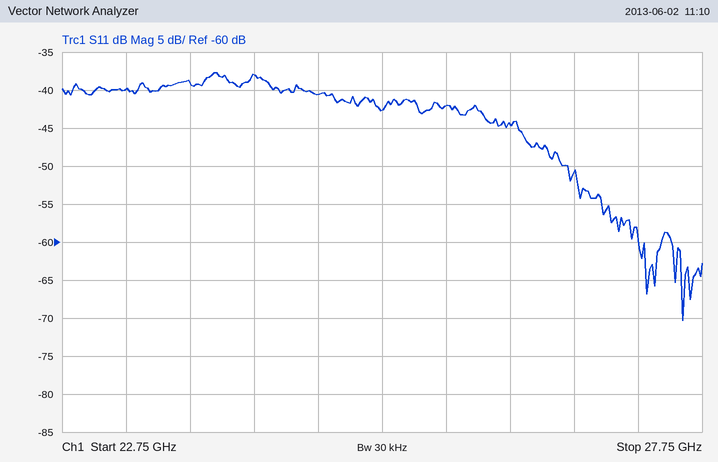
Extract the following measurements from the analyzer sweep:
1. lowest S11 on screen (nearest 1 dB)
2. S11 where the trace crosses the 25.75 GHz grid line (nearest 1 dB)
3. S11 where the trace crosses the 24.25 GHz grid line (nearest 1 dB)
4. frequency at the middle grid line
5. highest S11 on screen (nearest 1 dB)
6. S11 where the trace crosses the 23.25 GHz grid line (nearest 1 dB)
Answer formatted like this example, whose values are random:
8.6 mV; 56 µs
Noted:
-70 dB; -42 dB; -38 dB; 25.25 GHz; -38 dB; -40 dB
